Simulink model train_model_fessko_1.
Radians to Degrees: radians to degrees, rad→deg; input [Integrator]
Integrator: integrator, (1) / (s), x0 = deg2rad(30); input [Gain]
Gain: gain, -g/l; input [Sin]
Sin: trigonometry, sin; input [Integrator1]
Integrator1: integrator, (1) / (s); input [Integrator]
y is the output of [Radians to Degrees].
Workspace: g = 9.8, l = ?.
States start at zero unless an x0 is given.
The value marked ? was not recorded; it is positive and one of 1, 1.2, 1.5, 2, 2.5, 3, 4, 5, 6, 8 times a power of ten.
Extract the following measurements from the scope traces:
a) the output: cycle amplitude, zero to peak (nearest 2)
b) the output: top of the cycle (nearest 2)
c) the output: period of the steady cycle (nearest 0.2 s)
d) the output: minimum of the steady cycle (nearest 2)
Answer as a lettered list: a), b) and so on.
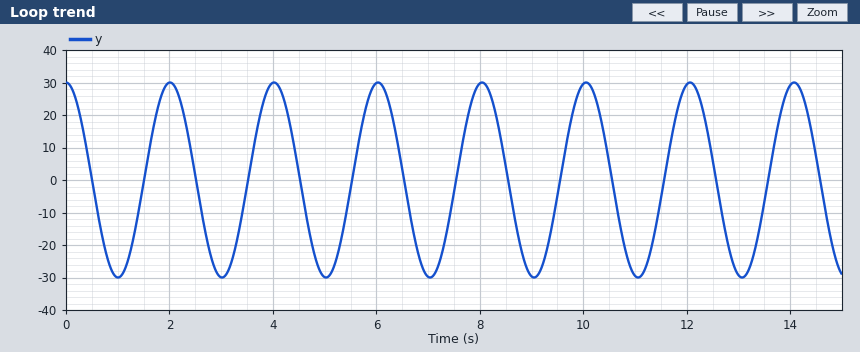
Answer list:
a) 30
b) 30
c) 2.0 s
d) -30
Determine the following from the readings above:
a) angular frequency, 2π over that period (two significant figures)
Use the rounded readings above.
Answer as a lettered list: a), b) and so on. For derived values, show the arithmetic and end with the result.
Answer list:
a) 2π / 2 = 3.1 rad/s
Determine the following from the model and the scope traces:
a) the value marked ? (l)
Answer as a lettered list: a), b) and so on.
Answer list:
a) 1
